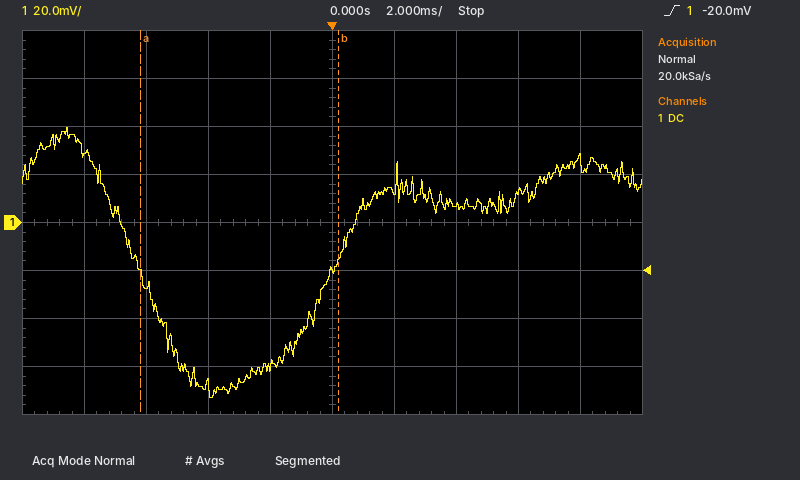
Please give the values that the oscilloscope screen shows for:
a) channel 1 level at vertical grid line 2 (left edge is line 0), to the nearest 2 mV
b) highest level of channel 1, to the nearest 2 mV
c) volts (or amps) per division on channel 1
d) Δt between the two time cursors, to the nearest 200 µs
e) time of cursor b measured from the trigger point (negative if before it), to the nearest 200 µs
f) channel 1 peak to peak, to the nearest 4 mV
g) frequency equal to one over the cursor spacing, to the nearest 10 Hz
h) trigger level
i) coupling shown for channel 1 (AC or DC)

-26 mV
40 mV
20 mV
6.4 ms
+200 µs
112 mV
160 Hz
-20.0 mV
DC
